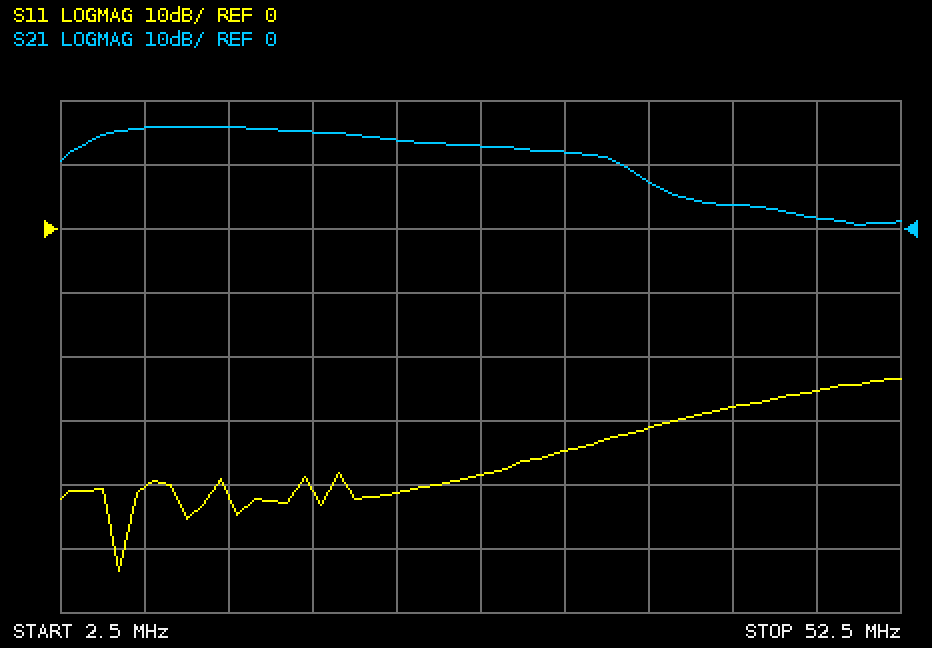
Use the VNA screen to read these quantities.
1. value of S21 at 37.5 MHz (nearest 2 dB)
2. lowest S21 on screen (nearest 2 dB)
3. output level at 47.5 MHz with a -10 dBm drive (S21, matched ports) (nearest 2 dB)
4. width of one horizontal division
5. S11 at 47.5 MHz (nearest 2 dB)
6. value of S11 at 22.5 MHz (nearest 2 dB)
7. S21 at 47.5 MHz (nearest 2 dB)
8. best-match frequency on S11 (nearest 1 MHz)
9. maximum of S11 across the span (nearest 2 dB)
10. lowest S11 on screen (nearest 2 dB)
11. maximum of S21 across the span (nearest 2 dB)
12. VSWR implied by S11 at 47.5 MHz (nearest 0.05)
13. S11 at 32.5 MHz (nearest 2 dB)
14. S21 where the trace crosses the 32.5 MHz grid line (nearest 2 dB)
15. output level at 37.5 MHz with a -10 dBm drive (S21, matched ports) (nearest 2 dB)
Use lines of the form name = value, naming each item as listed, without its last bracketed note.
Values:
value of S21 at 37.5 MHz = 8 dB
lowest S21 on screen = 0 dB
output level at 47.5 MHz with a -10 dBm drive (S21, matched ports) = -8 dBm
width of one horizontal division = 5 MHz
S11 at 47.5 MHz = -26 dB
value of S11 at 22.5 MHz = -42 dB
S21 at 47.5 MHz = 2 dB
best-match frequency on S11 = 6 MHz
maximum of S11 across the span = -24 dB
lowest S11 on screen = -54 dB
maximum of S21 across the span = 16 dB
VSWR implied by S11 at 47.5 MHz = 1.10
S11 at 32.5 MHz = -34 dB
S21 where the trace crosses the 32.5 MHz grid line = 12 dB
output level at 37.5 MHz with a -10 dBm drive (S21, matched ports) = -2 dBm
